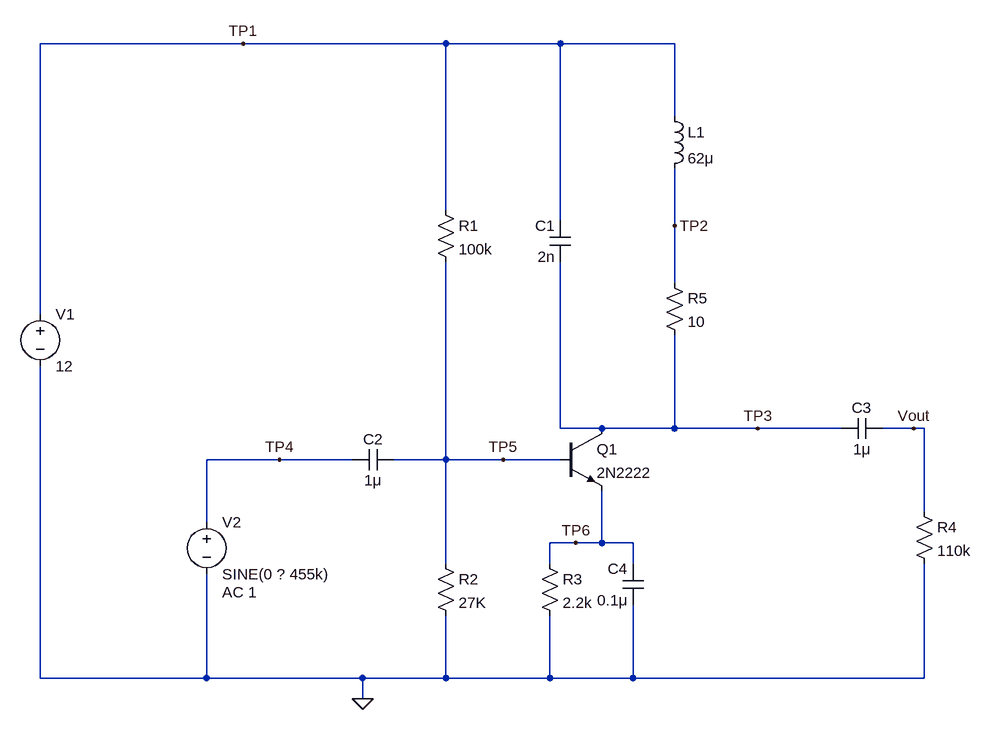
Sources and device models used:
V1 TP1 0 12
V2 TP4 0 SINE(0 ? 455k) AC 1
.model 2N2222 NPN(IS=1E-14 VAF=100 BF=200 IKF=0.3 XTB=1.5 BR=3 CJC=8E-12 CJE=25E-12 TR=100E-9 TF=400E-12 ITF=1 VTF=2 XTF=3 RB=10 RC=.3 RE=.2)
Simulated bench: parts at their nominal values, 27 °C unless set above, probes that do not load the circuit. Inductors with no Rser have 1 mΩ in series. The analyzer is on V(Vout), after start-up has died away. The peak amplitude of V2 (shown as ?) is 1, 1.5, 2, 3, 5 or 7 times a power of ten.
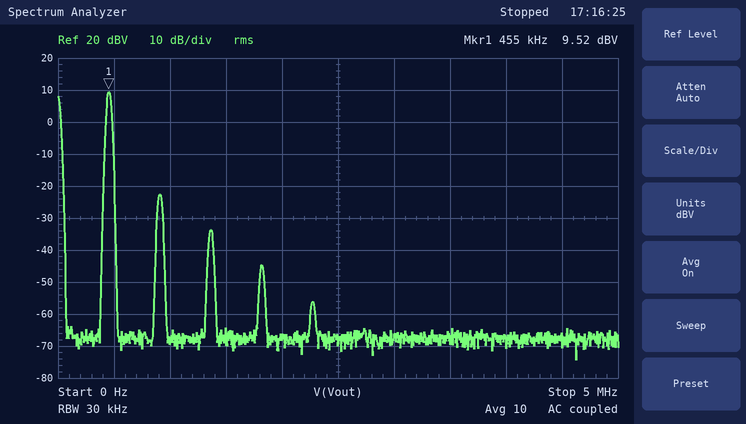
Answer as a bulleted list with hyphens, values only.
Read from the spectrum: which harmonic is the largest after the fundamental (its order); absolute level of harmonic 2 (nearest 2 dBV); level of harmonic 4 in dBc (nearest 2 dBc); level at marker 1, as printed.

- 2
- -22 dBV
- -54 dBc
- 9.52 dBV
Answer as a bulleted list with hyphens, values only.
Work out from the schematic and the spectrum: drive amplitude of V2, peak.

- 100 mV
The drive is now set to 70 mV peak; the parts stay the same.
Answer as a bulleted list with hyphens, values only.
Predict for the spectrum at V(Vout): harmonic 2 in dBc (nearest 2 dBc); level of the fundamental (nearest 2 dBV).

- -34 dBc
- 8 dBV
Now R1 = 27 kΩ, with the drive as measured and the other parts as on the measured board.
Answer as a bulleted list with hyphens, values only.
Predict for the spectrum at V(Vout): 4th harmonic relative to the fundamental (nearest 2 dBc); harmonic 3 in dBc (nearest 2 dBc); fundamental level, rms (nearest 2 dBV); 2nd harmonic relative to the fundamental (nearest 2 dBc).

- -32 dBc
- -32 dBc
- 14 dBV
- -42 dBc
